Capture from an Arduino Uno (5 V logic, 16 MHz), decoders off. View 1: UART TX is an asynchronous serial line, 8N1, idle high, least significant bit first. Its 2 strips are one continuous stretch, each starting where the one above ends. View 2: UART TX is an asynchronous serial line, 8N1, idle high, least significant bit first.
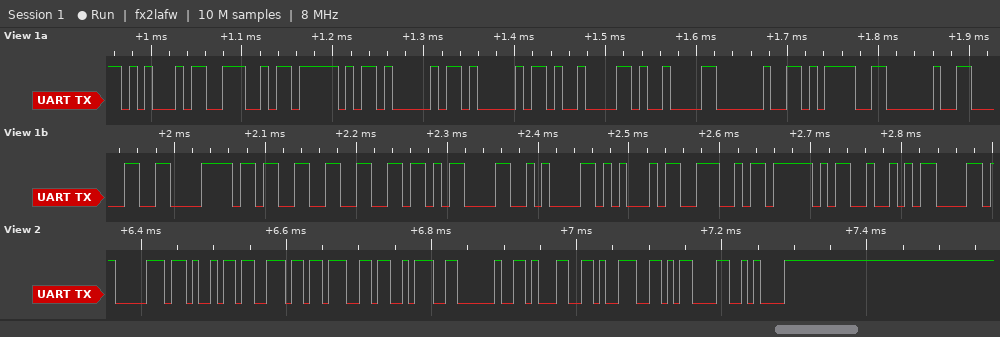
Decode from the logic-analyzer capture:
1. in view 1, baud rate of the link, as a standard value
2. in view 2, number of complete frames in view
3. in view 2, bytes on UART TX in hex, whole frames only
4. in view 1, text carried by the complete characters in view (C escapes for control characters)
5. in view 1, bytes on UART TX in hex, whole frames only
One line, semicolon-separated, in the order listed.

115200 baud; 10; 70 69 6E 67 3A 20 31 39 0D 0A; "EN_AA\t\t = 0x3f\r\nEN_R"; 45 4E 5F 41 41 09 09 20 3D 20 30 78 33 66 0D 0A 45 4E 5F 52
